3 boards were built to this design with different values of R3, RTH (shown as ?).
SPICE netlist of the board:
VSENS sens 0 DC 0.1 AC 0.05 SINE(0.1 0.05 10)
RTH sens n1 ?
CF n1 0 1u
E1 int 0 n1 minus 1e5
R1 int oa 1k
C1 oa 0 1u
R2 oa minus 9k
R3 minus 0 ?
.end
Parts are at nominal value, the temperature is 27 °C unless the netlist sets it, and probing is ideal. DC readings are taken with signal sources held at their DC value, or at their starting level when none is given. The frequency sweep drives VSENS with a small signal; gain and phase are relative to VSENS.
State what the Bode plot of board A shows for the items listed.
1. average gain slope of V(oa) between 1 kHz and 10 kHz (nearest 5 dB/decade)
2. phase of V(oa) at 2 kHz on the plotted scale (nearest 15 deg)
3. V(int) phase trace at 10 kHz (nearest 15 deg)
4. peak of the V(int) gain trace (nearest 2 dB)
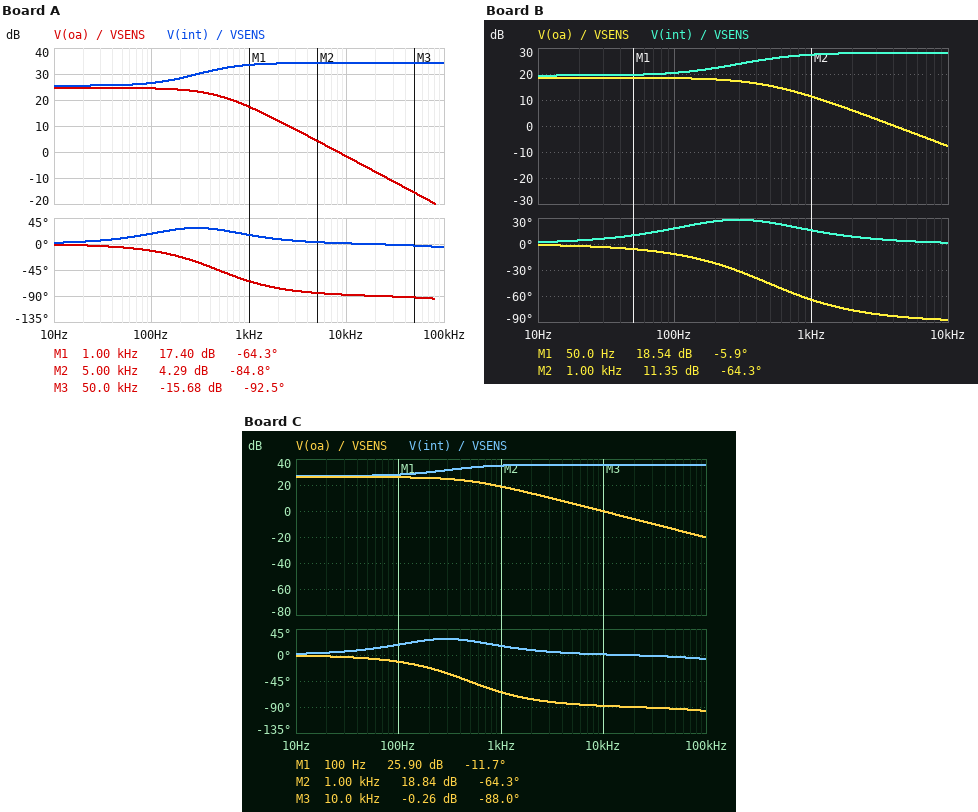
-20 dB/decade
-75 deg
0 deg
34 dB
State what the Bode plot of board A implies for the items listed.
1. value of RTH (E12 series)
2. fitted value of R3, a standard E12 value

330 Ω
560 Ω
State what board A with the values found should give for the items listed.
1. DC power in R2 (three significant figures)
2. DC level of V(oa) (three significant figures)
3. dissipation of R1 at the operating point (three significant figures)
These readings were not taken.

287 µW
1.71 V
31.9 µW
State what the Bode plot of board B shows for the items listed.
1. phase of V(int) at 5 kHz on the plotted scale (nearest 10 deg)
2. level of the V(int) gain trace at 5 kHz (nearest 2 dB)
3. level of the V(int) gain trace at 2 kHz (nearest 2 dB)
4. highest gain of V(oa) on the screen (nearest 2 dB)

0 deg
28 dB
28 dB
18 dB
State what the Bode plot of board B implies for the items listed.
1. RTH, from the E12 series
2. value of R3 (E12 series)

330 Ω
1.2 kΩ
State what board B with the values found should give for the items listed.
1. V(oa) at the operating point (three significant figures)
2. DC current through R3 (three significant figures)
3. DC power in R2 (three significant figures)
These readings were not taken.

850 mV
83.3 µA
62.5 µW
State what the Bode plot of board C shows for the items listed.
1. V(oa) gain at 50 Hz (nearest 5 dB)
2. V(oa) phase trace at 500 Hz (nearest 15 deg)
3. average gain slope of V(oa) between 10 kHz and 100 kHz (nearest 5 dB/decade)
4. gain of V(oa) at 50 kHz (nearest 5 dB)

25 dB
-45 deg
-20 dB/decade
-15 dB
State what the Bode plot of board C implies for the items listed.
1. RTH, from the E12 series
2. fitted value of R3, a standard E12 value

330 Ω
470 Ω
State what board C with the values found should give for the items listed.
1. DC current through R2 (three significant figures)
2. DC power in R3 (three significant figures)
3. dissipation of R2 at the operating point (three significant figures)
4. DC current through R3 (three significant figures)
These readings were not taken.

213 µA
21.3 µW
407 µW
213 µA
